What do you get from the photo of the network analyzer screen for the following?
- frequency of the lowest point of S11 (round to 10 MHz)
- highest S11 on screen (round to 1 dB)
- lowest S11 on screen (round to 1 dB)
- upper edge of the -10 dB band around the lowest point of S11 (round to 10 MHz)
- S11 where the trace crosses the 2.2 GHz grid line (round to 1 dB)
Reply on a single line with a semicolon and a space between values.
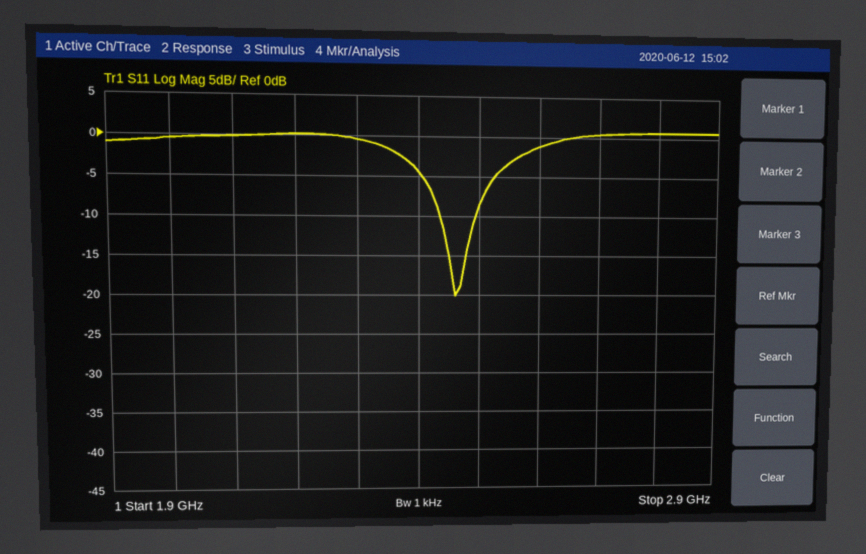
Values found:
2.46 GHz; 1 dB; -20 dB; 2.49 GHz; 0 dB
